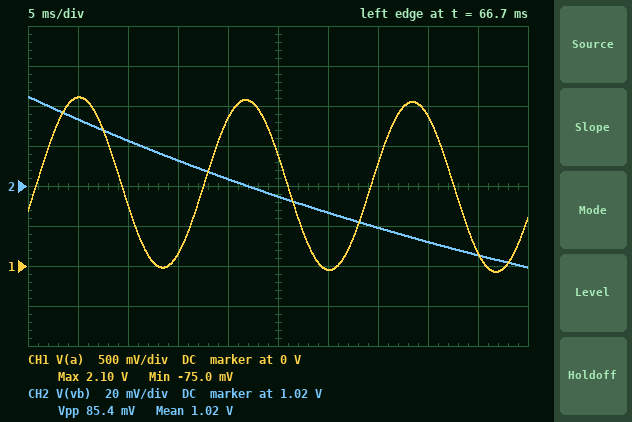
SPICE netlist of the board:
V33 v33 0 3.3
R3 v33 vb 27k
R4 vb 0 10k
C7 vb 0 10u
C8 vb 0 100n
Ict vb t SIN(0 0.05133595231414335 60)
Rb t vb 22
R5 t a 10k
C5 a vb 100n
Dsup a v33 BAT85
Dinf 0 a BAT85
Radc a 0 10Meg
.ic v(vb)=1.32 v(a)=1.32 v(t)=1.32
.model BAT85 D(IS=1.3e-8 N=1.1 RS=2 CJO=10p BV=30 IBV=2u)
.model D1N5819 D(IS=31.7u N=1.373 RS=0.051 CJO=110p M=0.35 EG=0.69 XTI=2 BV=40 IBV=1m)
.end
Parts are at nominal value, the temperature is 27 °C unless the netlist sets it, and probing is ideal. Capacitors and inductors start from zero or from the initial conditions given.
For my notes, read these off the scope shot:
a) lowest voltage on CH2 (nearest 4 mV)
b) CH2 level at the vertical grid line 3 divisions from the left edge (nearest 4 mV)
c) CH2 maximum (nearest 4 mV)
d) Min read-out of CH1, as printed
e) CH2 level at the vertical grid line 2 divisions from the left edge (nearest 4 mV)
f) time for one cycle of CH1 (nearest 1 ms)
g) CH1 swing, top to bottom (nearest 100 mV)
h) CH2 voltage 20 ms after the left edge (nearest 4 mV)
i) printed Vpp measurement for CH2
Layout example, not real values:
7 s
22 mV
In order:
980 mV
1.032 V
1.064 V
-75.0 mV
1.044 V
17 ms
2.2 V
1.024 V
85.4 mV
